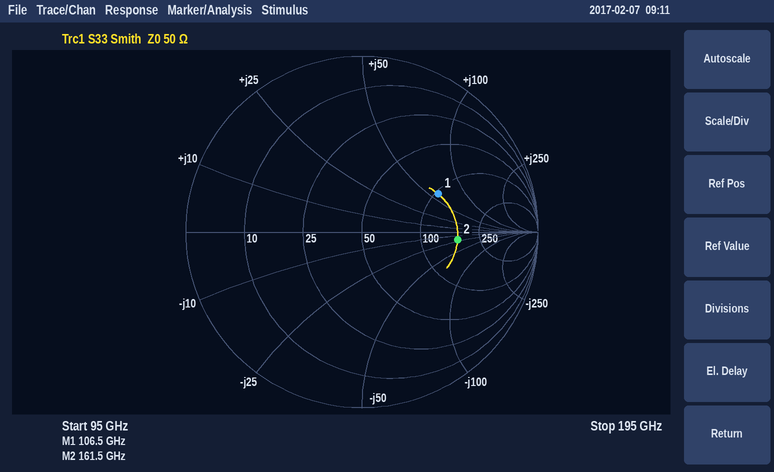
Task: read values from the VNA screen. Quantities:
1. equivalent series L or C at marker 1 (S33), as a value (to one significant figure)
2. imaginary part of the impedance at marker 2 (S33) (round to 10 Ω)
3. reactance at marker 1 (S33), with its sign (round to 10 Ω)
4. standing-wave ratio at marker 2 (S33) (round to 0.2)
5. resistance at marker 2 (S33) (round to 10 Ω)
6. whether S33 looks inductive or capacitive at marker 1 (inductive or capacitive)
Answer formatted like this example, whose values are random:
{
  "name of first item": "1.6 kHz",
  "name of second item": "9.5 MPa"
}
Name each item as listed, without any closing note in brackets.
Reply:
{
  "equivalent series L or C at marker 1 (S33), as a value": "90 pH",
  "imaginary part of the impedance at marker 2 (S33)": "-20 Ω",
  "reactance at marker 1 (S33), with its sign": "+60 Ω",
  "standing-wave ratio at marker 2 (S33)": "3.4",
  "resistance at marker 2 (S33)": "170 Ω",
  "whether S33 looks inductive or capacitive at marker 1": "inductive"
}
